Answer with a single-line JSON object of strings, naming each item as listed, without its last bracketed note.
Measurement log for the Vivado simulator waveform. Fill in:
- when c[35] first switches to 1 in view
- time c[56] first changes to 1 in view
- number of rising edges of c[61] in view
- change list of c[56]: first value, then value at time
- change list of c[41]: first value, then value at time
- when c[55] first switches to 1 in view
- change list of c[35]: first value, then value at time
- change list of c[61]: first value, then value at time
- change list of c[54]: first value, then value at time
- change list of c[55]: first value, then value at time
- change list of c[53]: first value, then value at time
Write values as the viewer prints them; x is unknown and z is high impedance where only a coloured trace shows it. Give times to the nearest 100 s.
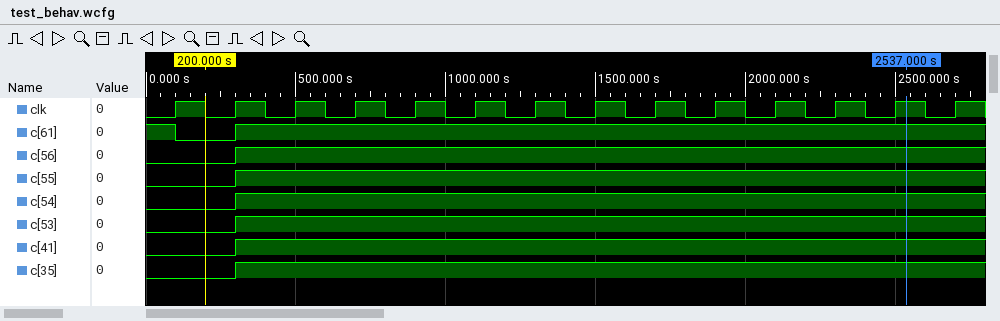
{"when c[35] first switches to 1 in view": "300 s", "time c[56] first changes to 1 in view": "300 s", "number of rising edges of c[61] in view": "1", "change list of c[56]: first value, then value at time": "0, 1 at 300 s", "change list of c[41]: first value, then value at time": "0, 1 at 300 s", "when c[55] first switches to 1 in view": "300 s", "change list of c[35]: first value, then value at time": "0, 1 at 300 s", "change list of c[61]: first value, then value at time": "1, 0 at 100 s, 1 at 300 s", "change list of c[54]: first value, then value at time": "0, 1 at 300 s", "change list of c[55]: first value, then value at time": "0, 1 at 300 s", "change list of c[53]: first value, then value at time": "0, 1 at 300 s"}
